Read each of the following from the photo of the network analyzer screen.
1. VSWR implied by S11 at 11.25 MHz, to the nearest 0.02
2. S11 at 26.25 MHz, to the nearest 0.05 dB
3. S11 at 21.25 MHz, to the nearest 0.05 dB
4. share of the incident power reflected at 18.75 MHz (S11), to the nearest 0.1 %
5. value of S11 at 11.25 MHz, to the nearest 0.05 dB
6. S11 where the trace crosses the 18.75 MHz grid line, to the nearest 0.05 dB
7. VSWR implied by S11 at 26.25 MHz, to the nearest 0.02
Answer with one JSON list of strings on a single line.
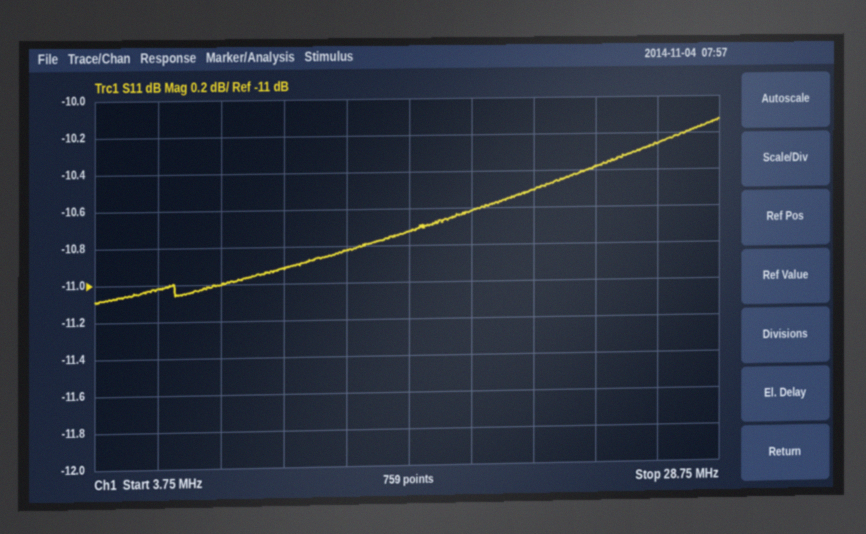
["1.80", "-10.25 dB", "-10.50 dB", "8.7 %", "-10.90 dB", "-10.60 dB", "1.88"]
